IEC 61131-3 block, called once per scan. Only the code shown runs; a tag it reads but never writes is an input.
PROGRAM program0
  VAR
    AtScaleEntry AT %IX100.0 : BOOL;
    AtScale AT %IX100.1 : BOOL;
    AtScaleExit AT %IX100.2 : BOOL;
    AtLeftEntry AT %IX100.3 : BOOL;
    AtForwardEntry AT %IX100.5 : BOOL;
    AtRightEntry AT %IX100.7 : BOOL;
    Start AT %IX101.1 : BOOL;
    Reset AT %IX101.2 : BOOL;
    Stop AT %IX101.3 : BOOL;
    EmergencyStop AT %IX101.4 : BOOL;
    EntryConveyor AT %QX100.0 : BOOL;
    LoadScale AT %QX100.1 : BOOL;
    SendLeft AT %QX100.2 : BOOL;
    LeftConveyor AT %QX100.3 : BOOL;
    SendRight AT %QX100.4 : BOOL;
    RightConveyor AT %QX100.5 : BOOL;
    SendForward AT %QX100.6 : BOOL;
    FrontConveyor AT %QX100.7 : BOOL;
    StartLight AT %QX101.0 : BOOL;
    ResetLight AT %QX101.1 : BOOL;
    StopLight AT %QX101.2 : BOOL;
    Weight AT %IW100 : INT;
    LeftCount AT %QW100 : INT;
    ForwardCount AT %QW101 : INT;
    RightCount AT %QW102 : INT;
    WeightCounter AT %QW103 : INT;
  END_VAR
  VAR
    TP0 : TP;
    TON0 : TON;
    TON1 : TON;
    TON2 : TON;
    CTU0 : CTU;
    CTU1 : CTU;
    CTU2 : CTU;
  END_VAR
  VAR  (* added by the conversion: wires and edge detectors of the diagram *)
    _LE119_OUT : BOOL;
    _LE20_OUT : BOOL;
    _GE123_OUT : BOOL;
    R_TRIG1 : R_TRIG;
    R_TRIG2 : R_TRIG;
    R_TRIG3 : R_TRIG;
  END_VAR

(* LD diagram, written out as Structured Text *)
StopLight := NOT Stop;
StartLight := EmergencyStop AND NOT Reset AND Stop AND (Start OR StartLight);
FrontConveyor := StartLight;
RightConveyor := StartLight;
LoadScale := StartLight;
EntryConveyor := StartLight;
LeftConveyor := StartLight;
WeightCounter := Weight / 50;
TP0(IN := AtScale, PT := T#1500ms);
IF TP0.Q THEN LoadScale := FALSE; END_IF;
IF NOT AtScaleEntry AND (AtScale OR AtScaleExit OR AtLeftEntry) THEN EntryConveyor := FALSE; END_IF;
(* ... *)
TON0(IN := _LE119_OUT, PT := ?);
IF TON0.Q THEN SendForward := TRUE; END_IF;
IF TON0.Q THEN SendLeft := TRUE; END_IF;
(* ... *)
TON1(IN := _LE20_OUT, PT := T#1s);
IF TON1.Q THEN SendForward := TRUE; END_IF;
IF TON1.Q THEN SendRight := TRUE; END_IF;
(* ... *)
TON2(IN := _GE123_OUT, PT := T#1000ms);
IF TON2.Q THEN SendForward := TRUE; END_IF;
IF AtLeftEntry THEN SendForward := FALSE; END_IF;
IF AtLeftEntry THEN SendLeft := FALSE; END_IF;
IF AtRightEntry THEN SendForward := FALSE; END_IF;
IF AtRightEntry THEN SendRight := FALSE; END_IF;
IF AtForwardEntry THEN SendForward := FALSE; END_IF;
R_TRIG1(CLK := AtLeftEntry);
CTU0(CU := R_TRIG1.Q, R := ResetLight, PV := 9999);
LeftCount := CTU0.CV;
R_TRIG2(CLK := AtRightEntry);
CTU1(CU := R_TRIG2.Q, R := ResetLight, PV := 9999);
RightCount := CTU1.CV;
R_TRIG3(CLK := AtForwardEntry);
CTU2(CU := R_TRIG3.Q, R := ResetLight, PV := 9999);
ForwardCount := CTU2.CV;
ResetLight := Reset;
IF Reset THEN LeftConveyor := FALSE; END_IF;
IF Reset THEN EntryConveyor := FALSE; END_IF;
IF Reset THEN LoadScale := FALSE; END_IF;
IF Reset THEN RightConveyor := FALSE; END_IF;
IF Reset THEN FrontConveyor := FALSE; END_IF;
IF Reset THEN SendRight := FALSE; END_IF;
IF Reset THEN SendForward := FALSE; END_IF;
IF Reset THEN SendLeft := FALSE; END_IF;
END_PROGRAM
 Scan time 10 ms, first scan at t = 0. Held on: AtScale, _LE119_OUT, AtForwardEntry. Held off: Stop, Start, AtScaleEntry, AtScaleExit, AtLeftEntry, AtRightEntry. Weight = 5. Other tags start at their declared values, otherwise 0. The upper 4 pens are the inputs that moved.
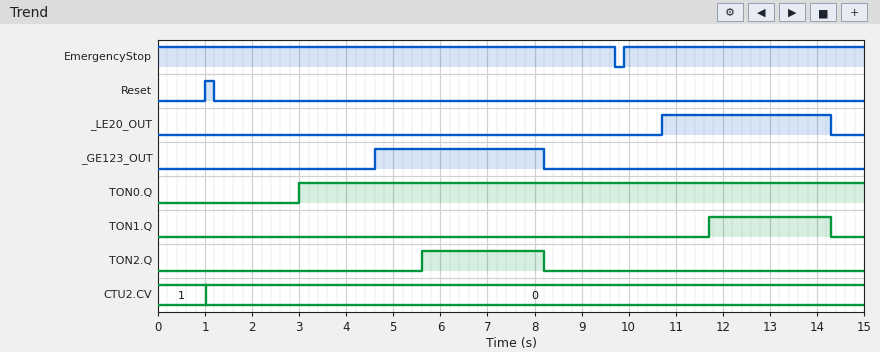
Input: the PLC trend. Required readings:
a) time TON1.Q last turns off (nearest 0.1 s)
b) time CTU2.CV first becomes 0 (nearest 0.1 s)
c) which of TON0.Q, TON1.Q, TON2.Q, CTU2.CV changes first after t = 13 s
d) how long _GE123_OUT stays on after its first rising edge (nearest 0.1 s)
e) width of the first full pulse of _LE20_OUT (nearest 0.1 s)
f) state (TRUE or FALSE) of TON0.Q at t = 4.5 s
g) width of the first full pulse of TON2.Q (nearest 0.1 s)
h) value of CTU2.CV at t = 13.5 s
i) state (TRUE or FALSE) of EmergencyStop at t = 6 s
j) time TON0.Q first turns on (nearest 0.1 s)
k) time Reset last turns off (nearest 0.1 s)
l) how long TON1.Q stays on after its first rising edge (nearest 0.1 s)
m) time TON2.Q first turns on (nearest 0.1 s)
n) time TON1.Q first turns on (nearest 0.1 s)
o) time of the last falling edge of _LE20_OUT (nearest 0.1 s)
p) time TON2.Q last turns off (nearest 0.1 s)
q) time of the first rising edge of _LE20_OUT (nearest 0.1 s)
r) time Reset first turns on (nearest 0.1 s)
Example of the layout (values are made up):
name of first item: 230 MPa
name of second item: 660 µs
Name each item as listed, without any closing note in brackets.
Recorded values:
time TON1.Q last turns off: 14.3 s
time CTU2.CV first becomes 0: 1.0 s
which of TON0.Q, TON1.Q, TON2.Q, CTU2.CV changes first after t = 13 s: TON1.Q
how long _GE123_OUT stays on after its first rising edge: 3.6 s
width of the first full pulse of _LE20_OUT: 3.6 s
state (TRUE or FALSE) of TON0.Q at t = 4.5 s: TRUE
width of the first full pulse of TON2.Q: 2.6 s
value of CTU2.CV at t = 13.5 s: 0
state (TRUE or FALSE) of EmergencyStop at t = 6 s: TRUE
time TON0.Q first turns on: 3.0 s
time Reset last turns off: 1.2 s
how long TON1.Q stays on after its first rising edge: 2.6 s
time TON2.Q first turns on: 5.6 s
time TON1.Q first turns on: 11.7 s
time of the last falling edge of _LE20_OUT: 14.3 s
time TON2.Q last turns off: 8.2 s
time of the first rising edge of _LE20_OUT: 10.7 s
time Reset first turns on: 1.0 s
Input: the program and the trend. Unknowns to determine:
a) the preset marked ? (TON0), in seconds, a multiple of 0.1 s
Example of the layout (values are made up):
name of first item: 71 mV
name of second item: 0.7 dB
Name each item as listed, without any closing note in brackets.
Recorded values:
the preset marked ? (TON0), in seconds, a multiple of 0.1 s: 3.0 s
